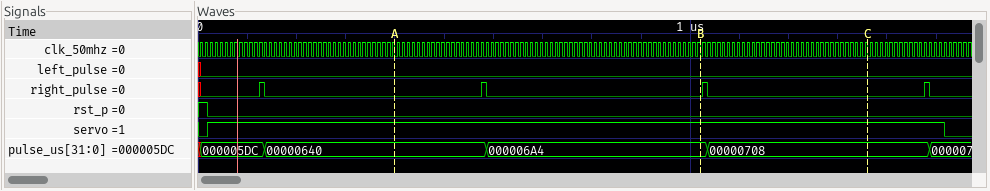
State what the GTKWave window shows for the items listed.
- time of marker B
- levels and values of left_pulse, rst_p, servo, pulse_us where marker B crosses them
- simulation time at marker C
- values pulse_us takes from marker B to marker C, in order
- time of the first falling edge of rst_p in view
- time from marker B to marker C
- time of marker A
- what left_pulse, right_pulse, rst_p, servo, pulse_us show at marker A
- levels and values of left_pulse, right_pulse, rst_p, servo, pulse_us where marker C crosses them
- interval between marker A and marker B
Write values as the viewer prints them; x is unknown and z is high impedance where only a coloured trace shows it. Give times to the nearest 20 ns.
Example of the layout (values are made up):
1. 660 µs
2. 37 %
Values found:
1. 1020 ns
2. left_pulse=0, rst_p=0, servo=1, pulse_us=000006A4
3. 1360 ns
4. 000006A4, 00000708
5. 20 ns
6. 340 ns
7. 400 ns
8. left_pulse=0, right_pulse=0, rst_p=0, servo=1, pulse_us=00000640
9. left_pulse=0, right_pulse=0, rst_p=0, servo=1, pulse_us=00000708
10. 620 ns
